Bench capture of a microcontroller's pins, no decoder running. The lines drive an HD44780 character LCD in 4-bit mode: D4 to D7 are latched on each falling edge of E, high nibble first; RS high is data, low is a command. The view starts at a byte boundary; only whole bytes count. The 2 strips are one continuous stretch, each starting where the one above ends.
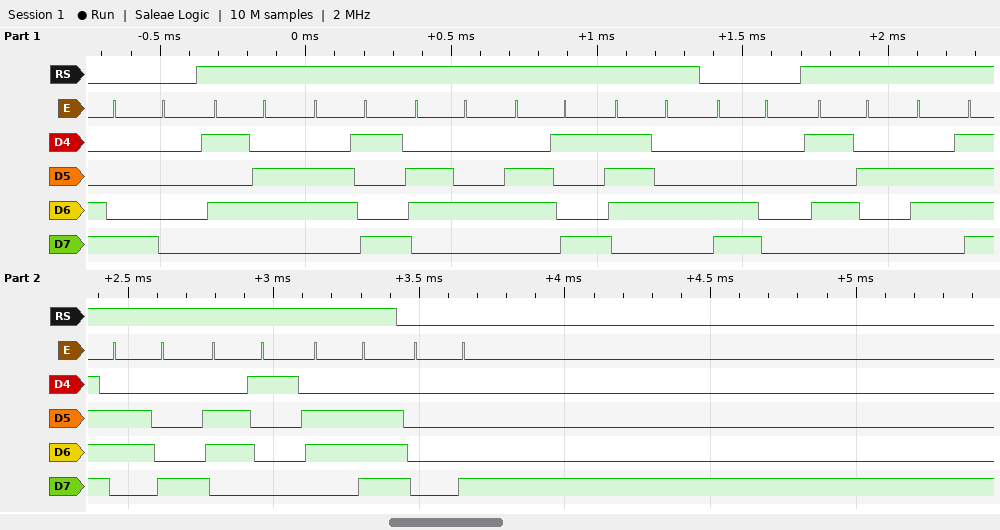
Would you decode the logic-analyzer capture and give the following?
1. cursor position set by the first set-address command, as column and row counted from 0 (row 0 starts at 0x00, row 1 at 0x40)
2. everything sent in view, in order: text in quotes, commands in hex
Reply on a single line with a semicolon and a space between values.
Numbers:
column 0, row 0; 0x80 "Vidit" 0xC0 "Rohan" 0x08
